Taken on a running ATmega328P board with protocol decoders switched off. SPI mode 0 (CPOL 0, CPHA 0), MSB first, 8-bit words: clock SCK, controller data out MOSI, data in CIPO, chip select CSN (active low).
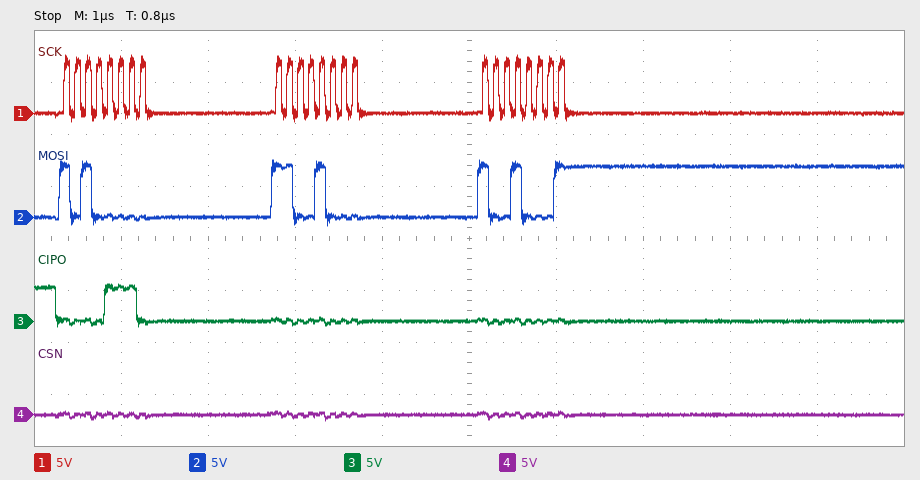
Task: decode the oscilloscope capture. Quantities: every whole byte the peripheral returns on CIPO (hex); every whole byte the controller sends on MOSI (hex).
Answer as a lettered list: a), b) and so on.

a) 0E 00 00
b) A0 C8 91
